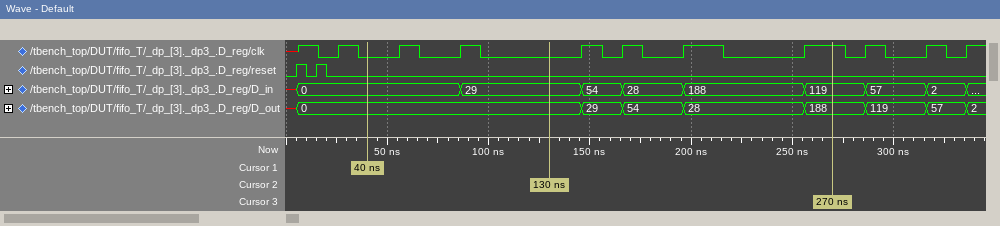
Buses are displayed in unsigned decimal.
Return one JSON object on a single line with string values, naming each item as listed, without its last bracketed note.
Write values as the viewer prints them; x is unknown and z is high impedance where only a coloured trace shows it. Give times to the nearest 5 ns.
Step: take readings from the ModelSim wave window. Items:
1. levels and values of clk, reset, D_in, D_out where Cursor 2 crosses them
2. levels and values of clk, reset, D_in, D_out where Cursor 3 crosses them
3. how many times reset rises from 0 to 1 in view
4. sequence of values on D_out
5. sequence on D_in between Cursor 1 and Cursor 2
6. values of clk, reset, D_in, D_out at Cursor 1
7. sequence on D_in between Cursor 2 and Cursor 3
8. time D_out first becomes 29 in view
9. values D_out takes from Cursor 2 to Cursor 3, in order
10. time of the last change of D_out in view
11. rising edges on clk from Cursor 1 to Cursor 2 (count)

{"levels and values of clk, reset, D_in, D_out where Cursor 2 crosses them": "clk=0, reset=0, D_in=29, D_out=0", "levels and values of clk, reset, D_in, D_out where Cursor 3 crosses them": "clk=1, reset=0, D_in=119, D_out=188", "how many times reset rises from 0 to 1 in view": "2", "sequence of values on D_out": "x, 0, 29, 54, 28, 188, 119, 57, 2", "sequence on D_in between Cursor 1 and Cursor 2": "0, 29", "values of clk, reset, D_in, D_out at Cursor 1": "clk=0, reset=0, D_in=0, D_out=0", "sequence on D_in between Cursor 2 and Cursor 3": "29, 54, 28, 188, 119", "time D_out first becomes 29 in view": "145 ns", "values D_out takes from Cursor 2 to Cursor 3, in order": "0, 29, 54, 28, 188", "time of the last change of D_out in view": "335 ns", "rising edges on clk from Cursor 1 to Cursor 2": "2"}
